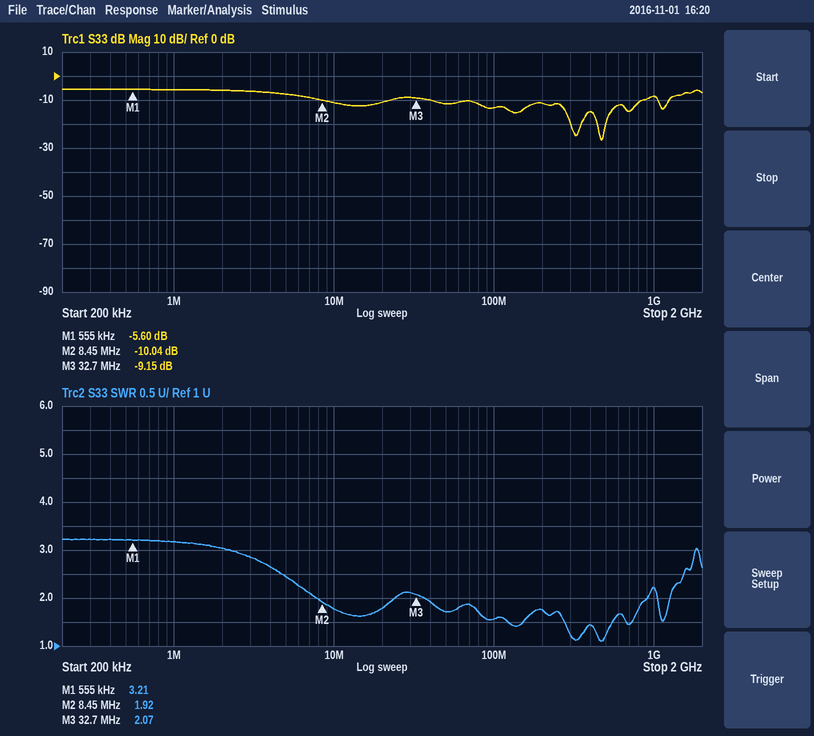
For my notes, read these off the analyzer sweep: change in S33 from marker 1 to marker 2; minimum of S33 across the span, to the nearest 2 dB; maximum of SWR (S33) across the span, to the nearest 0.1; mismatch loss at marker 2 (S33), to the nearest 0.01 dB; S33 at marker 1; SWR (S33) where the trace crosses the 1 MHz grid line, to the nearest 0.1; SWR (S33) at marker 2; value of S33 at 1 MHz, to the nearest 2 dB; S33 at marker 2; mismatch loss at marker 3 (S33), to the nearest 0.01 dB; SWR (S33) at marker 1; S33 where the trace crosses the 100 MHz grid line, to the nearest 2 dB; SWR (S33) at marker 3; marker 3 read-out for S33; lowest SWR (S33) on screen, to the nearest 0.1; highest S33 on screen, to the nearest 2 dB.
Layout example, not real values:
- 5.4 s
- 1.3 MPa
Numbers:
- -4.44 dB
- -26 dB
- 3.2
- 0.45 dB
- -5.60 dB
- 3.2
- 1.92
- -6 dB
- -10.04 dB
- 0.56 dB
- 3.21
- -14 dB
- 2.07
- -9.15 dB
- 1.1
- -6 dB
